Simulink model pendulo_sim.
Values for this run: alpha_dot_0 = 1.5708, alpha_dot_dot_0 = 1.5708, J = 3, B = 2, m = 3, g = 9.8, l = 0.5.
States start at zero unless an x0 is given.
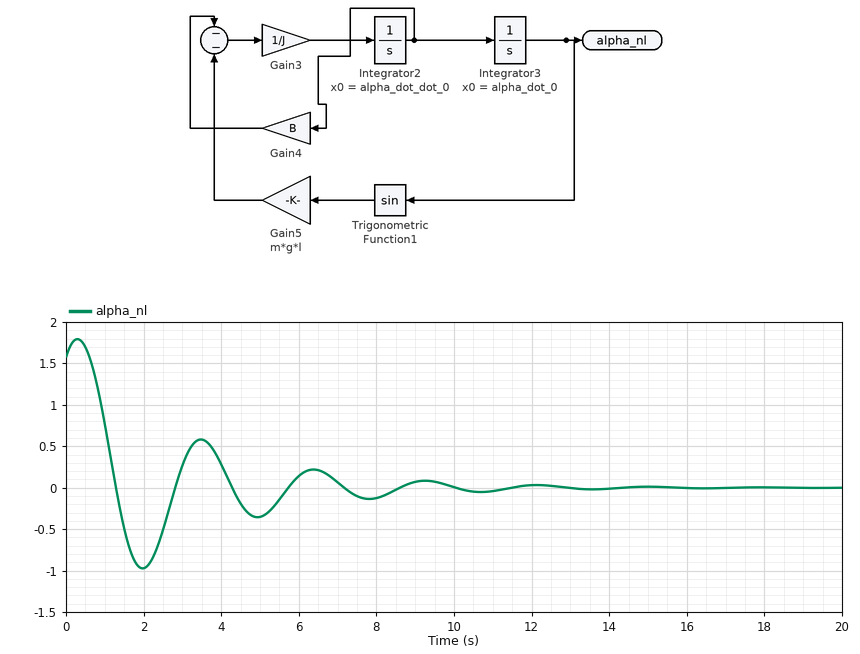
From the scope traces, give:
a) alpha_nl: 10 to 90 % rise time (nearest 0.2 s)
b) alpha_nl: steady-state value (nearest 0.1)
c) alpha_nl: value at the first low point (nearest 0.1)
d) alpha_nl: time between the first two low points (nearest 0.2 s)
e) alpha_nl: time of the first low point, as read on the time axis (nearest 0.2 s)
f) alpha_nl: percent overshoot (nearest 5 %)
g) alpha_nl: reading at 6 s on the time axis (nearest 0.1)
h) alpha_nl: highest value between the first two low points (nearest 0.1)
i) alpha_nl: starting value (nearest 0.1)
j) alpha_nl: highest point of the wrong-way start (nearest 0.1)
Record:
0.6 s
0.0
-1.0
3.0 s
2.0 s
60 %
0.1
0.6
1.6
1.8
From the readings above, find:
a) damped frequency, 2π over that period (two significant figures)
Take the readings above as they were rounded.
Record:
2.1 rad/s
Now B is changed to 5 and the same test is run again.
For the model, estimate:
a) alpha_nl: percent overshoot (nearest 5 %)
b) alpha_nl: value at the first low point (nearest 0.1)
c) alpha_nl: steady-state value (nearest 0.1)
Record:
25 %
-0.4
0.0
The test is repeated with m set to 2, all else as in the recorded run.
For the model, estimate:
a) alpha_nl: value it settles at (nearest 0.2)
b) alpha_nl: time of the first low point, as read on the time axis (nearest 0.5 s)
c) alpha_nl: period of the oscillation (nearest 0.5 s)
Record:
0.0
2.5 s
3.5 s
